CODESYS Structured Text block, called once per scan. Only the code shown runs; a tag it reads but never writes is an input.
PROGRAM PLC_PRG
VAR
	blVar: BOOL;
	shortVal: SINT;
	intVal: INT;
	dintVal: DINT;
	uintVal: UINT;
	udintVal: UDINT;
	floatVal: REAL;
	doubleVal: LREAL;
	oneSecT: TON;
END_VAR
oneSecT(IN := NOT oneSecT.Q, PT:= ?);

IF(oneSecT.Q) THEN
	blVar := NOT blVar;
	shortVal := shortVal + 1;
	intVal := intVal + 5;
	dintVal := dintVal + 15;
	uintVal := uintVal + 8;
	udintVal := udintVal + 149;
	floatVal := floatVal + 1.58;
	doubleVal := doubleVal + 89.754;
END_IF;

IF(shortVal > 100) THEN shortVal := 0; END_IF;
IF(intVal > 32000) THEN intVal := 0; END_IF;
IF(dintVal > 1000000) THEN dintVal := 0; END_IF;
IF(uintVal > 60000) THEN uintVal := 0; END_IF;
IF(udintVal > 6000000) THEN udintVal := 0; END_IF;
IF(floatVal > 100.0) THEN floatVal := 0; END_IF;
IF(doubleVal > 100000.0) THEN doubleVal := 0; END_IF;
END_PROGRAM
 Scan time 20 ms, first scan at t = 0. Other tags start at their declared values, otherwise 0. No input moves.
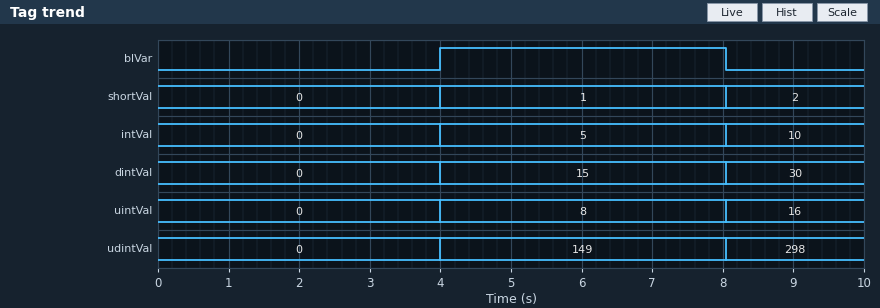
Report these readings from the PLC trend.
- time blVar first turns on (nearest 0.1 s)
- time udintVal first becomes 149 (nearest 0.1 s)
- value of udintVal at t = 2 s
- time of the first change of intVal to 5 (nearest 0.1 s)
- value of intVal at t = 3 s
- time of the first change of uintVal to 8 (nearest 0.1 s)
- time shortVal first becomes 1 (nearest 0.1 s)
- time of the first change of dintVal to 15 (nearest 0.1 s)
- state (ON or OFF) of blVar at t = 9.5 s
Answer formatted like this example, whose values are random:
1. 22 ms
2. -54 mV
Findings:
1. 4.0 s
2. 4.0 s
3. 0
4. 4.0 s
5. 0
6. 4.0 s
7. 4.0 s
8. 4.0 s
9. OFF
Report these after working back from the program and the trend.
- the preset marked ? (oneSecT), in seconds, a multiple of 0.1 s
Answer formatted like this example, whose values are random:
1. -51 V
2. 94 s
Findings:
1. 4.0 s
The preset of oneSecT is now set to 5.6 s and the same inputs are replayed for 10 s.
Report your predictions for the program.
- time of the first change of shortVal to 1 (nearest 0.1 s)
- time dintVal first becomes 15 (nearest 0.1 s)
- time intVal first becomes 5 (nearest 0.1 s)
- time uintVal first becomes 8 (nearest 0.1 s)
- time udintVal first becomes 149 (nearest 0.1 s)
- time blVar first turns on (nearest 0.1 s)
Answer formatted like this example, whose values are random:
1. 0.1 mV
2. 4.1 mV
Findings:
1. 5.6 s
2. 5.6 s
3. 5.6 s
4. 5.6 s
5. 5.6 s
6. 5.6 s
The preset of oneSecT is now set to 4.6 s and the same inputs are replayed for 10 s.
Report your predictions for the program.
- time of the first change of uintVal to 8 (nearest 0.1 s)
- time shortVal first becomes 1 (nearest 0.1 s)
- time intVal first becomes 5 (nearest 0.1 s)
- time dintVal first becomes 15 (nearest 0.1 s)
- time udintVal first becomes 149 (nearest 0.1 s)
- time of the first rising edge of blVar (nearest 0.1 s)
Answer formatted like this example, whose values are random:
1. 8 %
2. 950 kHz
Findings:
1. 4.6 s
2. 4.6 s
3. 4.6 s
4. 4.6 s
5. 4.6 s
6. 4.6 s
